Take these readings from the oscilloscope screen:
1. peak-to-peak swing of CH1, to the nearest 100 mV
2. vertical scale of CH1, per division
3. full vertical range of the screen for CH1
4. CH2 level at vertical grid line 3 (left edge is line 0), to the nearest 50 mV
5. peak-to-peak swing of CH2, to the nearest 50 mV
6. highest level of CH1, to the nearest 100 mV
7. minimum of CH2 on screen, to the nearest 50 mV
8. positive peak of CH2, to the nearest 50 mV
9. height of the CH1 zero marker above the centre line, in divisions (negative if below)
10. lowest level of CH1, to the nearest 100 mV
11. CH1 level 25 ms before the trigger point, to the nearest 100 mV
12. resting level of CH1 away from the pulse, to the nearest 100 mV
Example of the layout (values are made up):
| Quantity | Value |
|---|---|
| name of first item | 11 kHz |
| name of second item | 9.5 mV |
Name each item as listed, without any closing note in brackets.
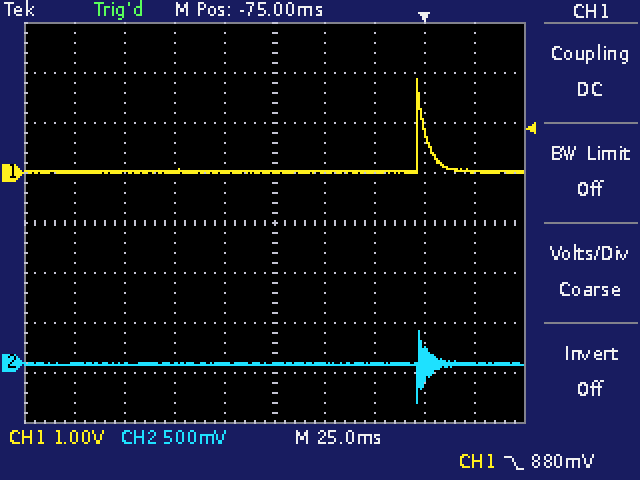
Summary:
| Quantity | Value |
|---|---|
| peak-to-peak swing of CH1, to the nearest 100 mV | 1.9 V |
| vertical scale of CH1, per division | 1 V |
| full vertical range of the screen for CH1 | 8 V |
| CH2 level at vertical grid line 3 (left edge is line 0), to the nearest 50 mV | 0 mV |
| peak-to-peak swing of CH2, to the nearest 50 mV | 700 mV |
| highest level of CH1, to the nearest 100 mV | 1.9 V |
| minimum of CH2 on screen, to the nearest 50 mV | -400 mV |
| positive peak of CH2, to the nearest 50 mV | 300 mV |
| height of the CH1 zero marker above the centre line, in divisions | +1.0 div |
| lowest level of CH1, to the nearest 100 mV | 0.0 V |
| CH1 level 25 ms before the trigger point, to the nearest 100 mV | 0.0 V |
| resting level of CH1 away from the pulse, to the nearest 100 mV | 0.0 V |
